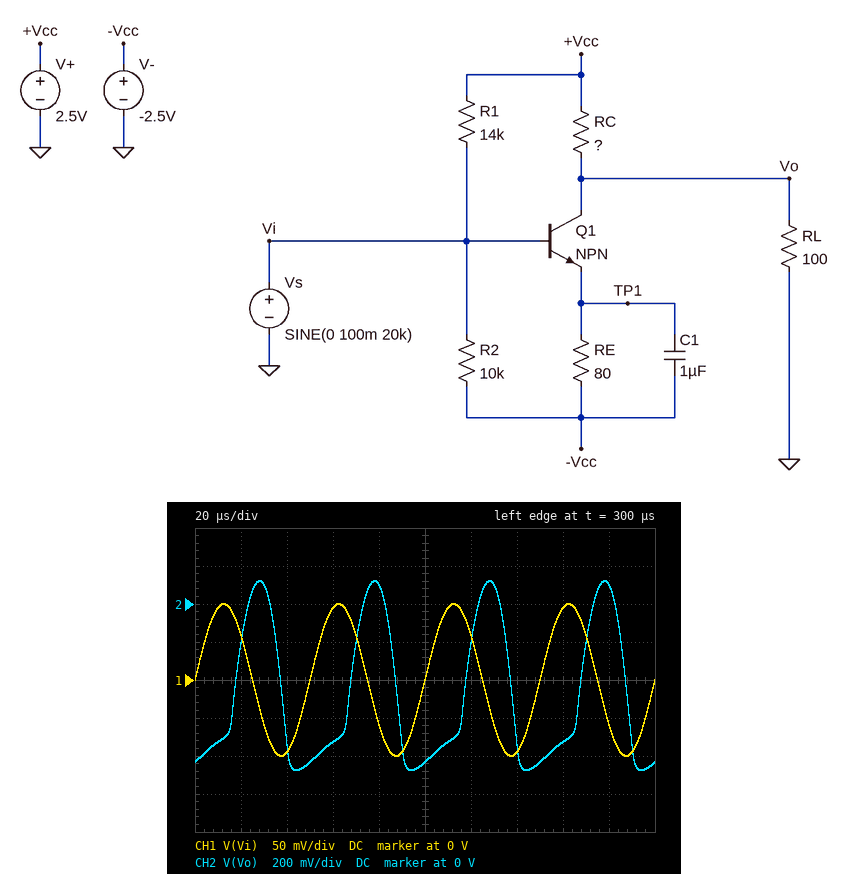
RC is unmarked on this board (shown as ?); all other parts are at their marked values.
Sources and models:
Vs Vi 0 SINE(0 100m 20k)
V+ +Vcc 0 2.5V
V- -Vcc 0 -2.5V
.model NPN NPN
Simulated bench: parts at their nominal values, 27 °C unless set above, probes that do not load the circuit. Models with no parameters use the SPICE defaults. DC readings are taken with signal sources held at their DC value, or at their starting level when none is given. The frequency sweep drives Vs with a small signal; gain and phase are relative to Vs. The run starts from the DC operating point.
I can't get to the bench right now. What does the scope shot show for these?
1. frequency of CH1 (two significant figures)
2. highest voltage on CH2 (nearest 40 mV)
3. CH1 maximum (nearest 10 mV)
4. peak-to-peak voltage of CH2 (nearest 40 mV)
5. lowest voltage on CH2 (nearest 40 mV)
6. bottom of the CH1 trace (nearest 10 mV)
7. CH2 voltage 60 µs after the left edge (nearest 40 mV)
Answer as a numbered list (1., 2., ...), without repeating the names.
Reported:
1. 20 kHz
2. 120 mV
3. 100 mV
4. 1.00 V
5. -880 mV
6. -100 mV
7. -720 mV
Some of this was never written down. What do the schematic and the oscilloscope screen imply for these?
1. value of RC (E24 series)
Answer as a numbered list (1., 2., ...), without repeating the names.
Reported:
1. 240 Ω
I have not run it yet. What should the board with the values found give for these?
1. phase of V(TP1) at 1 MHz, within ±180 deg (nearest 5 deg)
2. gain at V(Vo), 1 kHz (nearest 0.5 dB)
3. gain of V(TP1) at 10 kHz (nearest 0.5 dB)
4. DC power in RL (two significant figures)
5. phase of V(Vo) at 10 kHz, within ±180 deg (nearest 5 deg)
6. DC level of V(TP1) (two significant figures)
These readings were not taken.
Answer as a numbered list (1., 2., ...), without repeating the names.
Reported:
1. -85 deg
2. -3.0 dB
3. 0 dB
4. 4.9 mW
5. -105 deg
6. -850 mV
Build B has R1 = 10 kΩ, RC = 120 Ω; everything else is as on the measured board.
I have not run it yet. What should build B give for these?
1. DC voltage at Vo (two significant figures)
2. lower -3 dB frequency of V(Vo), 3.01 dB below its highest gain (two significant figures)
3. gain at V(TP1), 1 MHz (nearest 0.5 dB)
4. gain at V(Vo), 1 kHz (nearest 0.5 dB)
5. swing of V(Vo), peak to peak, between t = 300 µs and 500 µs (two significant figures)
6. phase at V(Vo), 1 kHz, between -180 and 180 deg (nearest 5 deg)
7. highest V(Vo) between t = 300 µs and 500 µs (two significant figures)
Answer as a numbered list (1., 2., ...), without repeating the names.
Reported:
1. 24 mV
2. 130 kHz
3. -18.0 dB
4. -2.5 dB
5. 1.3 V
6. -155 deg
7. 660 mV
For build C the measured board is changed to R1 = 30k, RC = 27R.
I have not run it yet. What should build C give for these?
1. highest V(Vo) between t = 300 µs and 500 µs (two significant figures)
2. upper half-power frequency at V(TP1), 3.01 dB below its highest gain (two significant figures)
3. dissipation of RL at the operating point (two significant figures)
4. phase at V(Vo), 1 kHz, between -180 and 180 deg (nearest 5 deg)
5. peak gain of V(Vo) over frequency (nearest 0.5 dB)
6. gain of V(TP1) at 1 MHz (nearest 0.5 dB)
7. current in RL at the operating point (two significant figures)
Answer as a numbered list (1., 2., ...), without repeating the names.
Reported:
1. 1.8 V
2. 130 kHz
3. 24 mW
4. -155 deg
5. 24.5 dB
6. -18.0 dB
7. 15 mA
